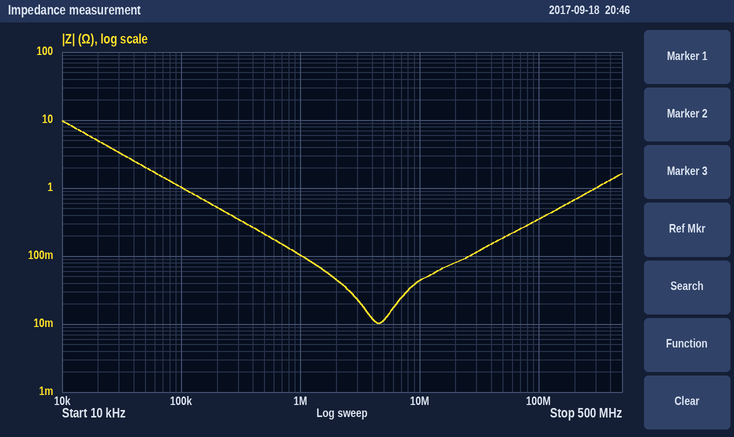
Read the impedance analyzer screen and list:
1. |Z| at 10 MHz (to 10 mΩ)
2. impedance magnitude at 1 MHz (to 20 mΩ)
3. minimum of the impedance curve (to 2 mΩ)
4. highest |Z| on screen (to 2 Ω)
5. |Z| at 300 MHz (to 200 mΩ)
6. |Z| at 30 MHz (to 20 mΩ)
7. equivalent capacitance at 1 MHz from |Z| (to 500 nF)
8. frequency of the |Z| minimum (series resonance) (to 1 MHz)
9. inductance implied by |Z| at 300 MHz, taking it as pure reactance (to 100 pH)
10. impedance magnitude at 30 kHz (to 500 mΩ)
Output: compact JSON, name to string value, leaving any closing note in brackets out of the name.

{"|Z| at 10 MHz": "40 mΩ", "impedance magnitude at 1 MHz": "100 mΩ", "minimum of the impedance curve": "10 mΩ", "highest |Z| on screen": "10 Ω", "|Z| at 300 MHz": "1.0 Ω", "|Z| at 30 MHz": "120 mΩ", "equivalent capacitance at 1 MHz from |Z|": "1.5 µF", "frequency of the |Z| minimum (series resonance)": "5 MHz", "inductance implied by |Z| at 300 MHz, taking it as pure reactance": "500 pH", "impedance magnitude at 30 kHz": "3.5 Ω"}
